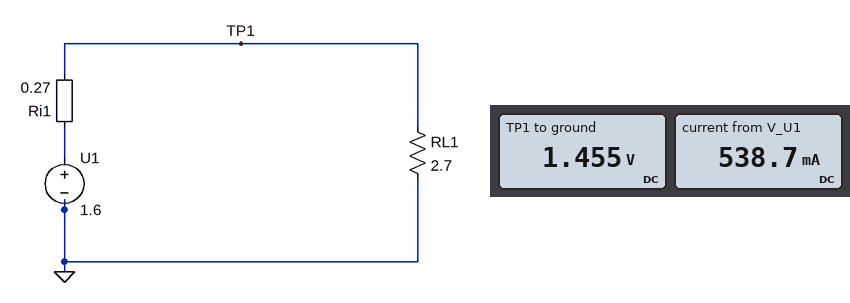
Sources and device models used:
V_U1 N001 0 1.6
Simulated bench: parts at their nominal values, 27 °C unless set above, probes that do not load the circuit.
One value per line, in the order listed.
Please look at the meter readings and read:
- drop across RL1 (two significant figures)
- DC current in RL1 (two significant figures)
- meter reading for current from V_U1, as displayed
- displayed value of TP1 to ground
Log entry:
1.5 V
540 mA
538.7 mA
1.455 V
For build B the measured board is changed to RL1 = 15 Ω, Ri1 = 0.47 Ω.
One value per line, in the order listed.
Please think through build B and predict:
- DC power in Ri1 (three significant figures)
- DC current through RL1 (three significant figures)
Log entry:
5.03 mW
103 mA
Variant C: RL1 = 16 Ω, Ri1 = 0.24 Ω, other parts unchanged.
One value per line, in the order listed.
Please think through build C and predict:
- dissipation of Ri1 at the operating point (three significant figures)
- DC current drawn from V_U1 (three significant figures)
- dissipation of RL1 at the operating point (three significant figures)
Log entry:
2.33 mW
98.5 mA
155 mW
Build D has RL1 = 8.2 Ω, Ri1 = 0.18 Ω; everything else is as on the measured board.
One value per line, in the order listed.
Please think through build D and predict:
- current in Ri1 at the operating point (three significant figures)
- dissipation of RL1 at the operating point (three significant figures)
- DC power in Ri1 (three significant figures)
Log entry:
191 mA
299 mW
6.56 mW
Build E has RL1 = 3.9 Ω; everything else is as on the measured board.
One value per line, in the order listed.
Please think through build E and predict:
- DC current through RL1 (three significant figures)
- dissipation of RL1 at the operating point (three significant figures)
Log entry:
384 mA
574 mW
